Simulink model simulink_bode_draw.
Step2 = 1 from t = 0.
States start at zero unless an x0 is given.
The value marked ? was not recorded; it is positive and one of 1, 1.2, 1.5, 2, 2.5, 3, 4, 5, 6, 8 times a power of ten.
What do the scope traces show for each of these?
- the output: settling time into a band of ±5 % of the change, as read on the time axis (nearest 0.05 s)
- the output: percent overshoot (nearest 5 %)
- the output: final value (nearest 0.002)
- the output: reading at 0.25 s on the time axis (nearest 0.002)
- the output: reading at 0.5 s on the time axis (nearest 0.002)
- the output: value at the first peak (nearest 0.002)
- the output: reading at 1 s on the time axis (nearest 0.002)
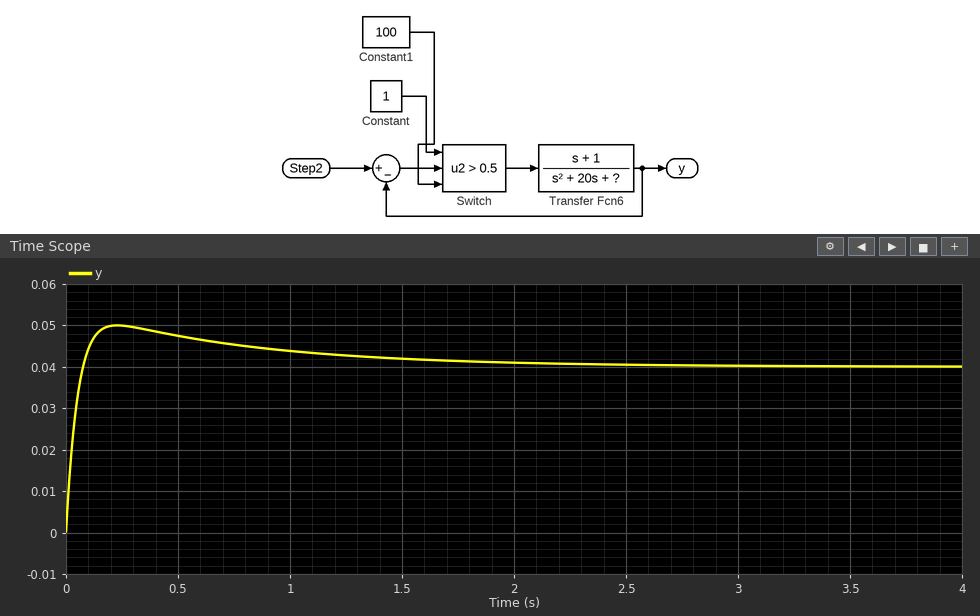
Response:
1.50 s
25 %
0.040
0.050
0.048
0.050
0.044
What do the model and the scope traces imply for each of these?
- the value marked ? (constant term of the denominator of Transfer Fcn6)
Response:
25
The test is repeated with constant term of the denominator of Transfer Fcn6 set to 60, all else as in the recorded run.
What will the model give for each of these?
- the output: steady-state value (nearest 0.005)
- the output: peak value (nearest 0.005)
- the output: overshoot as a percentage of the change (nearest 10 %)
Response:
0.015
0.045
160 %
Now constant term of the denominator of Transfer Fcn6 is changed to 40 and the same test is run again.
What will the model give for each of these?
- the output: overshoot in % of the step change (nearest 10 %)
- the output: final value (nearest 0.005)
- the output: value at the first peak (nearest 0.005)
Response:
90 %
0.025
0.045
